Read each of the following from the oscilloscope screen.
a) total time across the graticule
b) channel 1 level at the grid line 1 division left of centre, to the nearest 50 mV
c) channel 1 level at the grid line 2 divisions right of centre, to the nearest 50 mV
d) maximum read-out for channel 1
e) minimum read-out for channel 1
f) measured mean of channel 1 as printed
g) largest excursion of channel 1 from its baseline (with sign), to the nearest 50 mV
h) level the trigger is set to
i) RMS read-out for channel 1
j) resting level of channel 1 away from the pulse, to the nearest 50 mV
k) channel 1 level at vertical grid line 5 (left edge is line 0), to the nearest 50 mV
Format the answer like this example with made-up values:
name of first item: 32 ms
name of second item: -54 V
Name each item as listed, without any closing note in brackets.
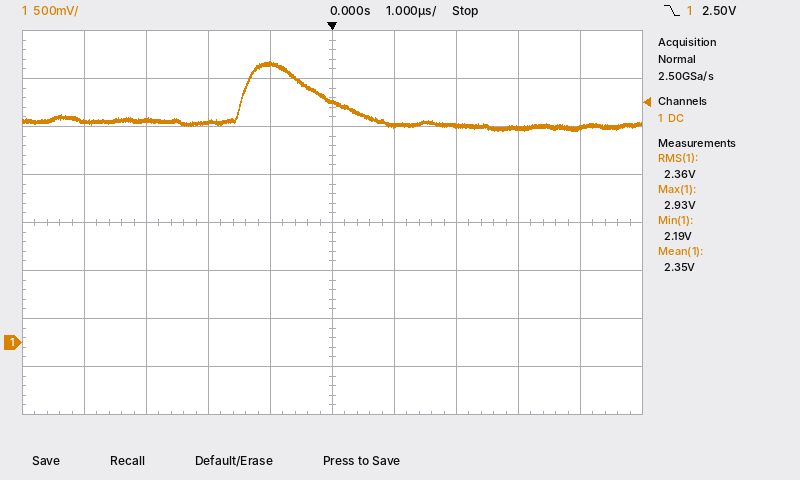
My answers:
total time across the graticule: 10 µs
channel 1 level at the grid line 1 division left of centre, to the nearest 50 mV: 2.90 V
channel 1 level at the grid line 2 divisions right of centre, to the nearest 50 mV: 2.25 V
maximum read-out for channel 1: 2.93 V
minimum read-out for channel 1: 2.19 V
measured mean of channel 1 as printed: 2.35 V
largest excursion of channel 1 from its baseline (with sign), to the nearest 50 mV: +650 mV
level the trigger is set to: 2.50 V
RMS read-out for channel 1: 2.36 V
resting level of channel 1 away from the pulse, to the nearest 50 mV: 2.30 V
channel 1 level at vertical grid line 5 (left edge is line 0), to the nearest 50 mV: 2.50 V
